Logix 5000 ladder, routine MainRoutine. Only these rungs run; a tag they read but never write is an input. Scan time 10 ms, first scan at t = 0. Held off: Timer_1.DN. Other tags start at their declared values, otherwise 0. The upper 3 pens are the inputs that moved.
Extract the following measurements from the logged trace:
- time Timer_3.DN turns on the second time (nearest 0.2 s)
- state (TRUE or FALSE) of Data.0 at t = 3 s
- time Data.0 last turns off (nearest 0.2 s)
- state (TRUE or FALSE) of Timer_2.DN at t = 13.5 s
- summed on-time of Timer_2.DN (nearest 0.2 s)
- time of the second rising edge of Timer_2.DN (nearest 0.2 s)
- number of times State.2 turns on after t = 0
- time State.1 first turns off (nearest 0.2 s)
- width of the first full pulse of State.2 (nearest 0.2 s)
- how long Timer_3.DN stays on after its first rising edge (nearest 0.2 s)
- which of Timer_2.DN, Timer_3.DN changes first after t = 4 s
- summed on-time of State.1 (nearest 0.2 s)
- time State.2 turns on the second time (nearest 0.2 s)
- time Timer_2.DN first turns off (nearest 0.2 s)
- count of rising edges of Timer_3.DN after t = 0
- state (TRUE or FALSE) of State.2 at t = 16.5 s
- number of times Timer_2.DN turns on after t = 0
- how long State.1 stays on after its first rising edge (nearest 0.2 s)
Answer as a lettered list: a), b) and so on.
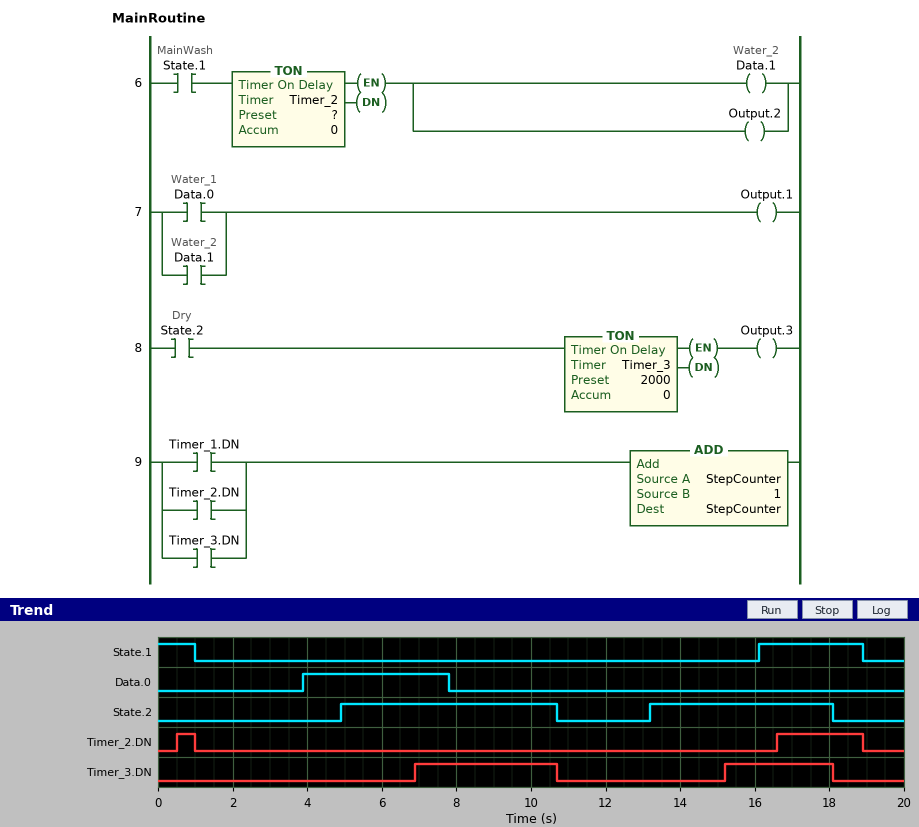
a) 15.2 s
b) FALSE
c) 7.8 s
d) FALSE
e) 2.8 s
f) 16.6 s
g) 2
h) 1.0 s
i) 5.8 s
j) 3.8 s
k) Timer_3.DN
l) 3.8 s
m) 13.2 s
n) 1.0 s
o) 2
p) TRUE
q) 2
r) 2.8 s
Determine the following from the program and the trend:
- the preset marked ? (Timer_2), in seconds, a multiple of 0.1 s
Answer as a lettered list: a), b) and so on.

a) 0.5 s
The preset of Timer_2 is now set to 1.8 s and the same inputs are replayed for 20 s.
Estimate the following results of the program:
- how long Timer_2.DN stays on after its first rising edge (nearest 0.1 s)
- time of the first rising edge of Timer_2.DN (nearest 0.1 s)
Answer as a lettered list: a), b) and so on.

a) 1.0 s
b) 17.9 s
